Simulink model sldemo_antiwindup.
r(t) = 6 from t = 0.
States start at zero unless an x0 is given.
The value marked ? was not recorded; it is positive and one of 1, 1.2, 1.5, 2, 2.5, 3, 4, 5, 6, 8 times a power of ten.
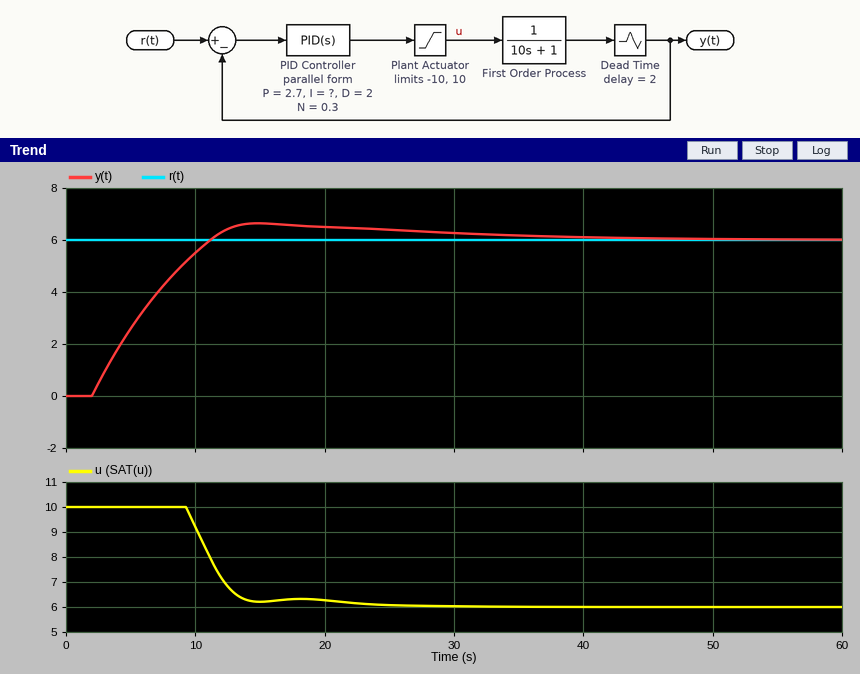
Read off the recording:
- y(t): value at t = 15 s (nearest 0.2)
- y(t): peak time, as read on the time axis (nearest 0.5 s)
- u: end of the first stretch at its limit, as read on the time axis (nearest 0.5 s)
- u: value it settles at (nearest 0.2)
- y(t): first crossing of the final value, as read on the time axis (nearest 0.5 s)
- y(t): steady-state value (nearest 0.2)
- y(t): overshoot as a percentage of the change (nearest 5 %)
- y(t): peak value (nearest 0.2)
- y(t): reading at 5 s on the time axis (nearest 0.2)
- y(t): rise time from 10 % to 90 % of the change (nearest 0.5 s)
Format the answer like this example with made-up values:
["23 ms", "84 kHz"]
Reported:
["6.6", "15.0 s", "9.5 s", "6.0", "11.0 s", "6.0", "10 %", "6.6", "2.6", "7.0 s"]
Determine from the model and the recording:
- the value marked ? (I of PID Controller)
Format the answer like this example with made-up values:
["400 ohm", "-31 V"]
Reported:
["0.25"]
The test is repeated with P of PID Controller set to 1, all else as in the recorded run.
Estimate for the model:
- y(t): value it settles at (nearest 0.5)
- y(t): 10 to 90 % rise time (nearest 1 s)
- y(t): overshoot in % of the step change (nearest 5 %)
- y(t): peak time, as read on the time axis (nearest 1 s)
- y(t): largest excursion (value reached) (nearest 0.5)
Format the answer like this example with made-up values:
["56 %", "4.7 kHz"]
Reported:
["6.0", "8 s", "15 %", "20 s", "7.0"]
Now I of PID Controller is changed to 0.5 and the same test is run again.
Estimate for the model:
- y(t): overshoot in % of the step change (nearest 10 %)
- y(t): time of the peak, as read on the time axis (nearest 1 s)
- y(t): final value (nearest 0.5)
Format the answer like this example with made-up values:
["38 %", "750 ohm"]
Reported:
["40 %", "20 s", "6.0"]
